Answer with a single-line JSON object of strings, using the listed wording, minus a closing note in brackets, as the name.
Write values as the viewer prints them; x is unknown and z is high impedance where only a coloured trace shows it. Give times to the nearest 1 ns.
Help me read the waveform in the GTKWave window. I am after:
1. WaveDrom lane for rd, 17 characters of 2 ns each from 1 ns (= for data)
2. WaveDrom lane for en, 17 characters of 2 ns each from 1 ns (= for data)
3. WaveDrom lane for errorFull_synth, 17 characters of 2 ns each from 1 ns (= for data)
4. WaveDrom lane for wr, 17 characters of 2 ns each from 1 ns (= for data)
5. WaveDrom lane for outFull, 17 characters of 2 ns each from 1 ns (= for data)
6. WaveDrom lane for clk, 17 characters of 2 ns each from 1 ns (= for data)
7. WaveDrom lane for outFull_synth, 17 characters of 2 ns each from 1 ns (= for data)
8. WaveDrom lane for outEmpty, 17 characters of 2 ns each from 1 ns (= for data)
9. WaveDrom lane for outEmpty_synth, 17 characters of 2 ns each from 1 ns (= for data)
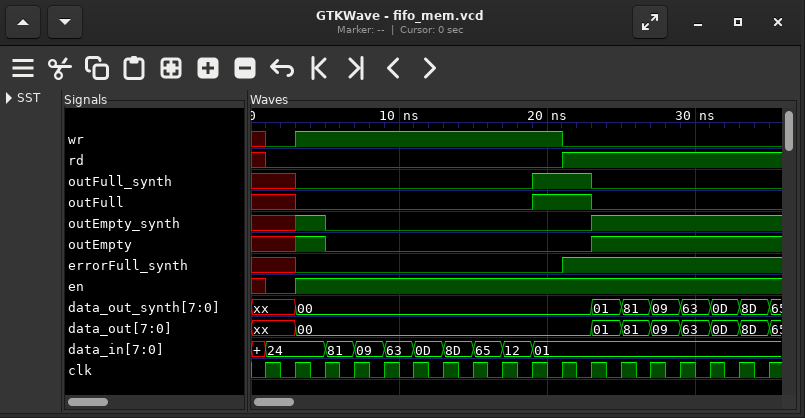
{"WaveDrom lane for rd, 17 characters of 2 ns each from 1 ns": "{name: 'rd', wave: '0.........1......'}", "WaveDrom lane for en, 17 characters of 2 ns each from 1 ns": "{name: 'en', wave: '01...............'}", "WaveDrom lane for errorFull_synth, 17 characters of 2 ns each from 1 ns": "{name: 'errorFull_synth', wave: 'x0........1......'}", "WaveDrom lane for wr, 17 characters of 2 ns each from 1 ns": "{name: 'wr', wave: '01........0......'}", "WaveDrom lane for outFull, 17 characters of 2 ns each from 1 ns": "{name: 'outFull', wave: 'x0.......1.0.....'}", "WaveDrom lane for clk, 17 characters of 2 ns each from 1 ns": "{name: 'clk', wave: 'p................'}", "WaveDrom lane for outFull_synth, 17 characters of 2 ns each from 1 ns": "{name: 'outFull_synth', wave: 'x0.......1.0.....'}", "WaveDrom lane for outEmpty, 17 characters of 2 ns each from 1 ns": "{name: 'outEmpty', wave: 'x10........1.....'}", "WaveDrom lane for outEmpty_synth, 17 characters of 2 ns each from 1 ns": "{name: 'outEmpty_synth', wave: 'x10........1.....'}"}
